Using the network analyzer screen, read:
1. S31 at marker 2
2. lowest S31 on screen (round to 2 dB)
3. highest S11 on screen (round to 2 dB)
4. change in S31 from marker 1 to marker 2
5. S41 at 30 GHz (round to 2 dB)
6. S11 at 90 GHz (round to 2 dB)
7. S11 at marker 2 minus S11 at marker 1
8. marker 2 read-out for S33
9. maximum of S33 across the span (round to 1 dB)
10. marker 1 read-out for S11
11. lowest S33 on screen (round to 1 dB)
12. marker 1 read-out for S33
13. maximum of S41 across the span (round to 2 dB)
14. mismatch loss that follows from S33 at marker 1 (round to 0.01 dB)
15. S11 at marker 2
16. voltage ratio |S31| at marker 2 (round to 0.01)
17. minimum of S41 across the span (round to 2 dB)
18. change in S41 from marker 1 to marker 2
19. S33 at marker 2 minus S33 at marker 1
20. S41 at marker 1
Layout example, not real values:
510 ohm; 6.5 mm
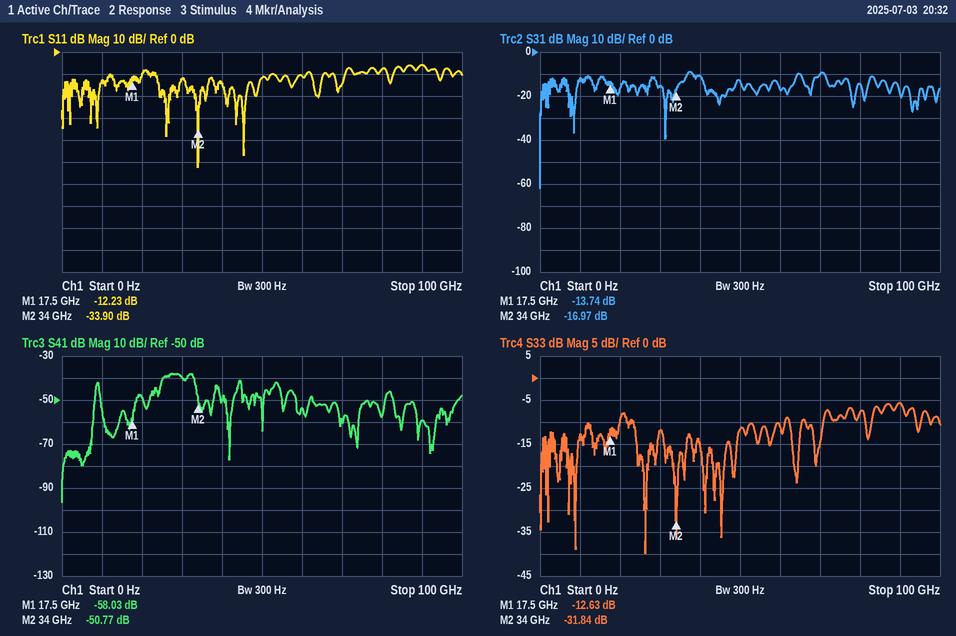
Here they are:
-16.97 dB; -62 dB; -6 dB; -3.23 dB; -40 dB; -6 dB; -21.67 dB; -31.84 dB; -6 dB; -12.23 dB; -40 dB; -12.63 dB; -38 dB; 0.24 dB; -33.90 dB; 0.14; -96 dB; 7.26 dB; -19.21 dB; -58.03 dB
